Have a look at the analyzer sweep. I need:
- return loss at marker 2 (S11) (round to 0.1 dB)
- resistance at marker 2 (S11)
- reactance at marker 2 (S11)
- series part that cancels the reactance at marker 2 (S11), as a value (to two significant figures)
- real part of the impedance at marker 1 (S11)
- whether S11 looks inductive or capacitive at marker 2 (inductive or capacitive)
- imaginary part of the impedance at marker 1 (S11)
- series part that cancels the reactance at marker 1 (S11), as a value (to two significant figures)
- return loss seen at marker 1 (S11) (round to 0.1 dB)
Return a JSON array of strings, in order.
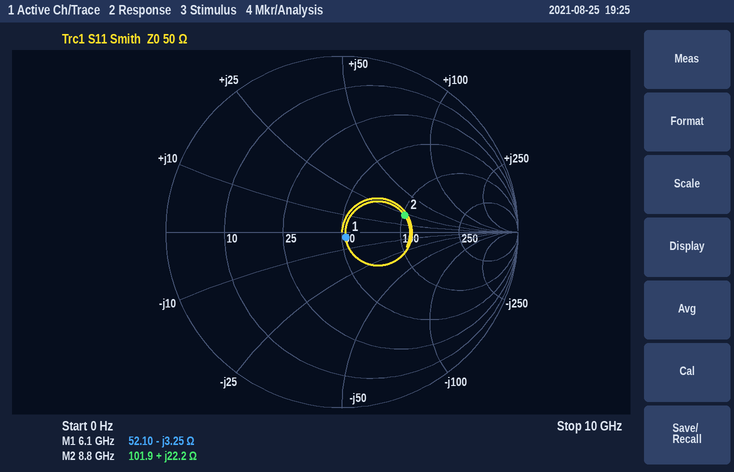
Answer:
["8.7 dB", "101.9 Ω", "+22.2 Ω", "810 fF", "52.10 Ω", "inductive", "-3.25 Ω", "85 pH", "28.4 dB"]
